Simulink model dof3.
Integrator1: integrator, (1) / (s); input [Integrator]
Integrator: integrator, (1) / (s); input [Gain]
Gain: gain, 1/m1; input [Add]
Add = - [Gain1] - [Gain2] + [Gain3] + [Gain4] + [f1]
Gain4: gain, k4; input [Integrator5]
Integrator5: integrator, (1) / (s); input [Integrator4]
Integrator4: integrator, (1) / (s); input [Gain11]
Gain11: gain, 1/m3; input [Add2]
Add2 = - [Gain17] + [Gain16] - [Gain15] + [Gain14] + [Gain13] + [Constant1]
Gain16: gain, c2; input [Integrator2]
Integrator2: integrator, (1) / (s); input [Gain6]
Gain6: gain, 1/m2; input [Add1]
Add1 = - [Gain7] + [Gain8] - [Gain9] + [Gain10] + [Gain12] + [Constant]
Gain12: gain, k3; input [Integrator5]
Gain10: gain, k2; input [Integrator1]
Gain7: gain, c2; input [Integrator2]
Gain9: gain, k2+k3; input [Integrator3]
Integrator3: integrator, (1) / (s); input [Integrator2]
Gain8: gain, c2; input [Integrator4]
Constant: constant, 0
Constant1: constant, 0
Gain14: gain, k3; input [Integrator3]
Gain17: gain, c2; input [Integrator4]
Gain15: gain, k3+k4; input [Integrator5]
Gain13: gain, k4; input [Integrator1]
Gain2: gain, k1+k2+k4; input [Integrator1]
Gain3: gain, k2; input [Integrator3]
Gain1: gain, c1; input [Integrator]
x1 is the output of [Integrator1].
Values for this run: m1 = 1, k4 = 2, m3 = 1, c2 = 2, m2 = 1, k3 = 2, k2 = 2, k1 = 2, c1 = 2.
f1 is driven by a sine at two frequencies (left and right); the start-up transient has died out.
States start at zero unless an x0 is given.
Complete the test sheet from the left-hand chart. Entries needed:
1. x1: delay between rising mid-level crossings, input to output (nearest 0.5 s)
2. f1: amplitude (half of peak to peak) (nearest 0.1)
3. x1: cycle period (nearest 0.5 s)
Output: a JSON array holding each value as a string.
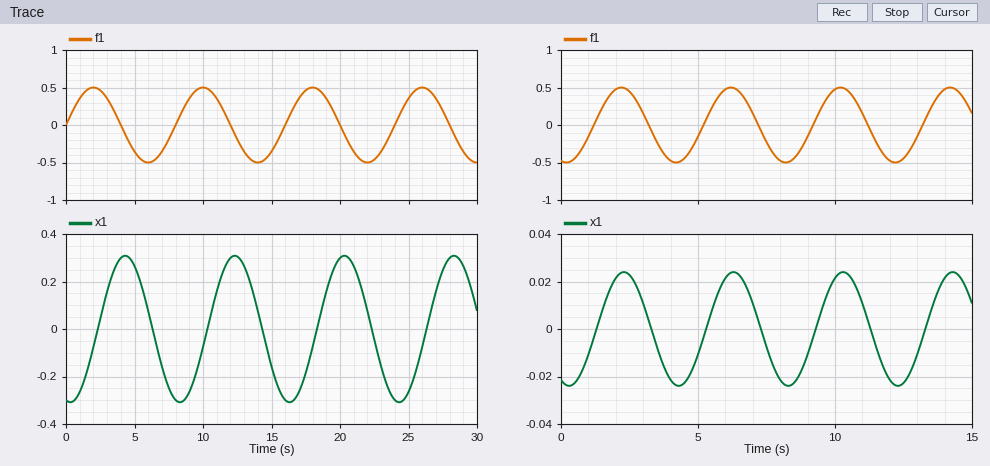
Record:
["2.5 s", "0.5", "8.0 s"]
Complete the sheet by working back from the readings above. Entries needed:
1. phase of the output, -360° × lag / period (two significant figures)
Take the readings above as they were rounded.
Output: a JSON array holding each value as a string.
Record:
["-110°"]
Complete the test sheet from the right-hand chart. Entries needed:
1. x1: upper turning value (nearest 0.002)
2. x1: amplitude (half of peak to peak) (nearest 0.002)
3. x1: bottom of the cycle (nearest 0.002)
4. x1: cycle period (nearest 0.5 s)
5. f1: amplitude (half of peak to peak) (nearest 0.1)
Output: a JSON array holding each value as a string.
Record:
["0.024", "0.024", "-0.024", "4.0 s", "0.5"]
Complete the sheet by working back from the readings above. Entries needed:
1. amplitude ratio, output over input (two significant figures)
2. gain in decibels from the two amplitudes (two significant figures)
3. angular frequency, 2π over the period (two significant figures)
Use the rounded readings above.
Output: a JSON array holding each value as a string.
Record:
["0.048", "-26 dB", "1.6 rad/s"]
